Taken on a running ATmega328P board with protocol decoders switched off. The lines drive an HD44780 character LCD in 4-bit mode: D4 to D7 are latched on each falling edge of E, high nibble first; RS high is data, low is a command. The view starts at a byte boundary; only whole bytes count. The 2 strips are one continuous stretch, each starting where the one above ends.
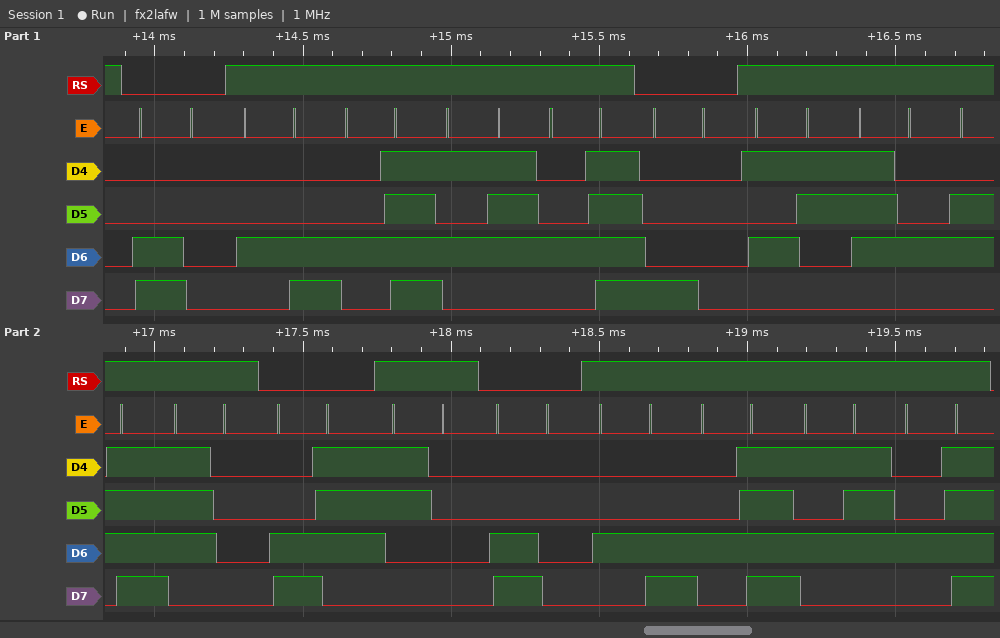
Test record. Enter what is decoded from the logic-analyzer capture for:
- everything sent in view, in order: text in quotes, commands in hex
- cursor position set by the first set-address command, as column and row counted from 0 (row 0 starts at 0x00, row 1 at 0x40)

0xC0 "LOWO" 0x80 "Stop" 0xC7 "0" 0xC0 "LOWO"
column 0, row 1
